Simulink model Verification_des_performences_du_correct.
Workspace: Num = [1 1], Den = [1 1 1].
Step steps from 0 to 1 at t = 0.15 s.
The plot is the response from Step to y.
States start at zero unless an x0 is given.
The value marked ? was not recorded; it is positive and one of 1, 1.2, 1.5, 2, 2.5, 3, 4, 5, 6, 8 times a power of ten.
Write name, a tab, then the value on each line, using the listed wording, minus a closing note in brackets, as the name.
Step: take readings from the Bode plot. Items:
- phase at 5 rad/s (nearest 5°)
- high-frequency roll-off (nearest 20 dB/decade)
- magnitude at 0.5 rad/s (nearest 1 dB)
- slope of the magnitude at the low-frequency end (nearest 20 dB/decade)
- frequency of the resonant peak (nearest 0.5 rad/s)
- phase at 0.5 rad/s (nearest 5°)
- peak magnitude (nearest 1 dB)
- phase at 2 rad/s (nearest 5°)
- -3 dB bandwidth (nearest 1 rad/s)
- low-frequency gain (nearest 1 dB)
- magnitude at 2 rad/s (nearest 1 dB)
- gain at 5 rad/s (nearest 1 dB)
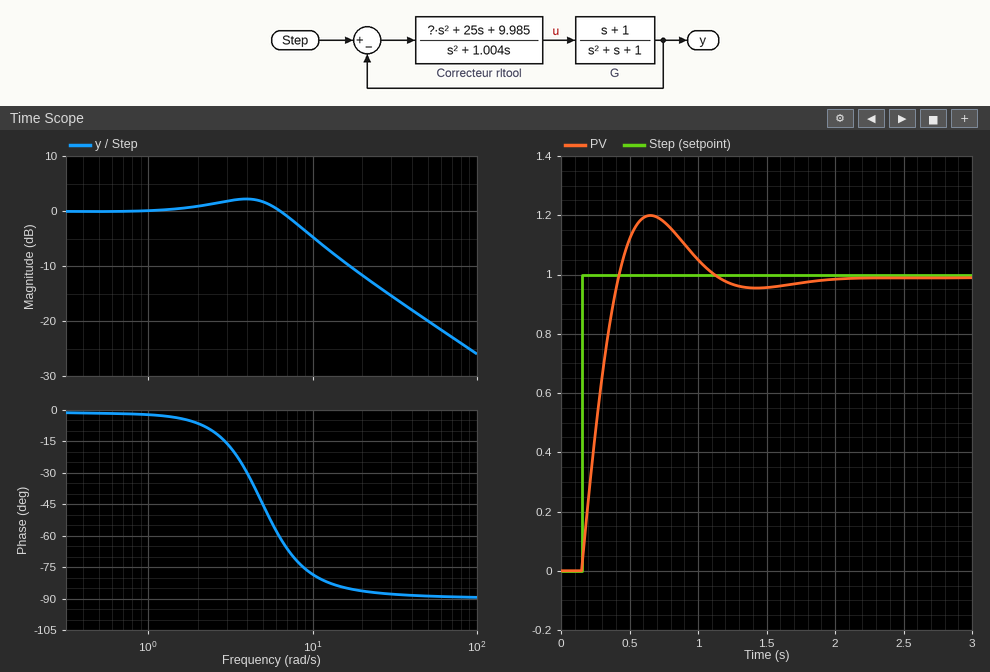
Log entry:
phase at 5 rad/s	-45°
high-frequency roll-off	-20 dB/decade
magnitude at 0.5 rad/s	0 dB
slope of the magnitude at the low-frequency end	0 dB/decade
frequency of the resonant peak	4.0 rad/s
phase at 0.5 rad/s	0°
peak magnitude	2 dB
phase at 2 rad/s	-5°
-3 dB bandwidth	9 rad/s
low-frequency gain	0 dB
magnitude at 2 rad/s	1 dB
gain at 5 rad/s	2 dB
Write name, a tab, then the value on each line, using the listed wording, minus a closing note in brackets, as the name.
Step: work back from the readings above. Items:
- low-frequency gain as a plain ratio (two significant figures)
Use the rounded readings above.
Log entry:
low-frequency gain as a plain ratio	1.0
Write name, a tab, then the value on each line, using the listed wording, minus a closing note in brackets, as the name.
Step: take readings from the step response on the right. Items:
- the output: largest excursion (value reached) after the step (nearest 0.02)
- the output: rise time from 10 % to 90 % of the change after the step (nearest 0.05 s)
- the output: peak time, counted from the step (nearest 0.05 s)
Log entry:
the output: largest excursion (value reached) after the step	1.20
the output: rise time from 10 % to 90 % of the change after the step	0.20 s
the output: peak time, counted from the step	0.50 s
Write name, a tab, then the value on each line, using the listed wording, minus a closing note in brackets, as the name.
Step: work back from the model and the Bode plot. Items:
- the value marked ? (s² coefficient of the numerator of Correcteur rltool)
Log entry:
the value marked ?	5
